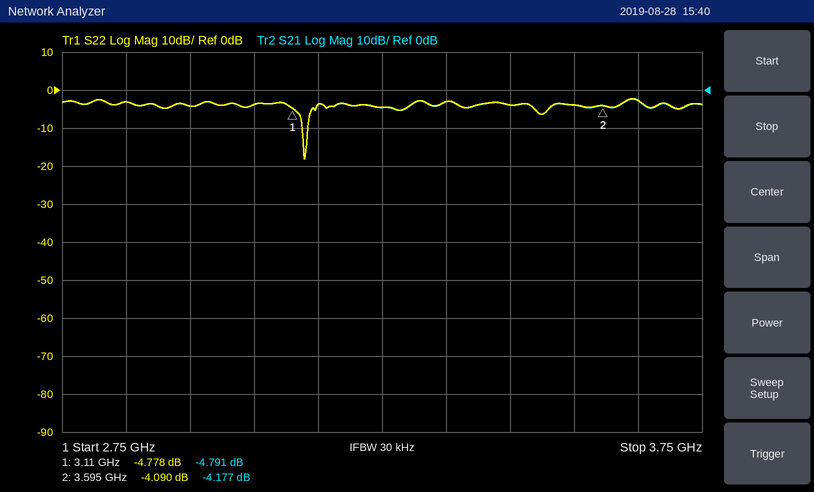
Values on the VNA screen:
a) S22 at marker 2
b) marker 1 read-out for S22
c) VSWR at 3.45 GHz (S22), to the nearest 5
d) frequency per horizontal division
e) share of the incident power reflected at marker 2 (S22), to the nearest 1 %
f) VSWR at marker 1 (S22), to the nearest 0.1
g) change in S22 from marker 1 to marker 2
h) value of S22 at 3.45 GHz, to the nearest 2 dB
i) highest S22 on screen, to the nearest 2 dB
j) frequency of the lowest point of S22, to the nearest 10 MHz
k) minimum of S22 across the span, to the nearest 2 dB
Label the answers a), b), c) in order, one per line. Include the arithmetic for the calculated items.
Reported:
a) -4.090 dB
b) -4.778 dB
c) |Γ| = 10^(-4/20) = 0.6310; VSWR = (1 + 0.6310)/(1 − 0.6310) ≈ 4.42, so 5 to the nearest 5
d) 100 MHz
e) 10^(-4.09/10) ≈ 39 %
f) (1 + 0.5769)/(1 − 0.5769) ≈ 3.7
g) -4.09 − (-4.778) = 0.688 dB
h) -4 dB
i) -2 dB
j) 3.13 GHz
k) -18 dB
